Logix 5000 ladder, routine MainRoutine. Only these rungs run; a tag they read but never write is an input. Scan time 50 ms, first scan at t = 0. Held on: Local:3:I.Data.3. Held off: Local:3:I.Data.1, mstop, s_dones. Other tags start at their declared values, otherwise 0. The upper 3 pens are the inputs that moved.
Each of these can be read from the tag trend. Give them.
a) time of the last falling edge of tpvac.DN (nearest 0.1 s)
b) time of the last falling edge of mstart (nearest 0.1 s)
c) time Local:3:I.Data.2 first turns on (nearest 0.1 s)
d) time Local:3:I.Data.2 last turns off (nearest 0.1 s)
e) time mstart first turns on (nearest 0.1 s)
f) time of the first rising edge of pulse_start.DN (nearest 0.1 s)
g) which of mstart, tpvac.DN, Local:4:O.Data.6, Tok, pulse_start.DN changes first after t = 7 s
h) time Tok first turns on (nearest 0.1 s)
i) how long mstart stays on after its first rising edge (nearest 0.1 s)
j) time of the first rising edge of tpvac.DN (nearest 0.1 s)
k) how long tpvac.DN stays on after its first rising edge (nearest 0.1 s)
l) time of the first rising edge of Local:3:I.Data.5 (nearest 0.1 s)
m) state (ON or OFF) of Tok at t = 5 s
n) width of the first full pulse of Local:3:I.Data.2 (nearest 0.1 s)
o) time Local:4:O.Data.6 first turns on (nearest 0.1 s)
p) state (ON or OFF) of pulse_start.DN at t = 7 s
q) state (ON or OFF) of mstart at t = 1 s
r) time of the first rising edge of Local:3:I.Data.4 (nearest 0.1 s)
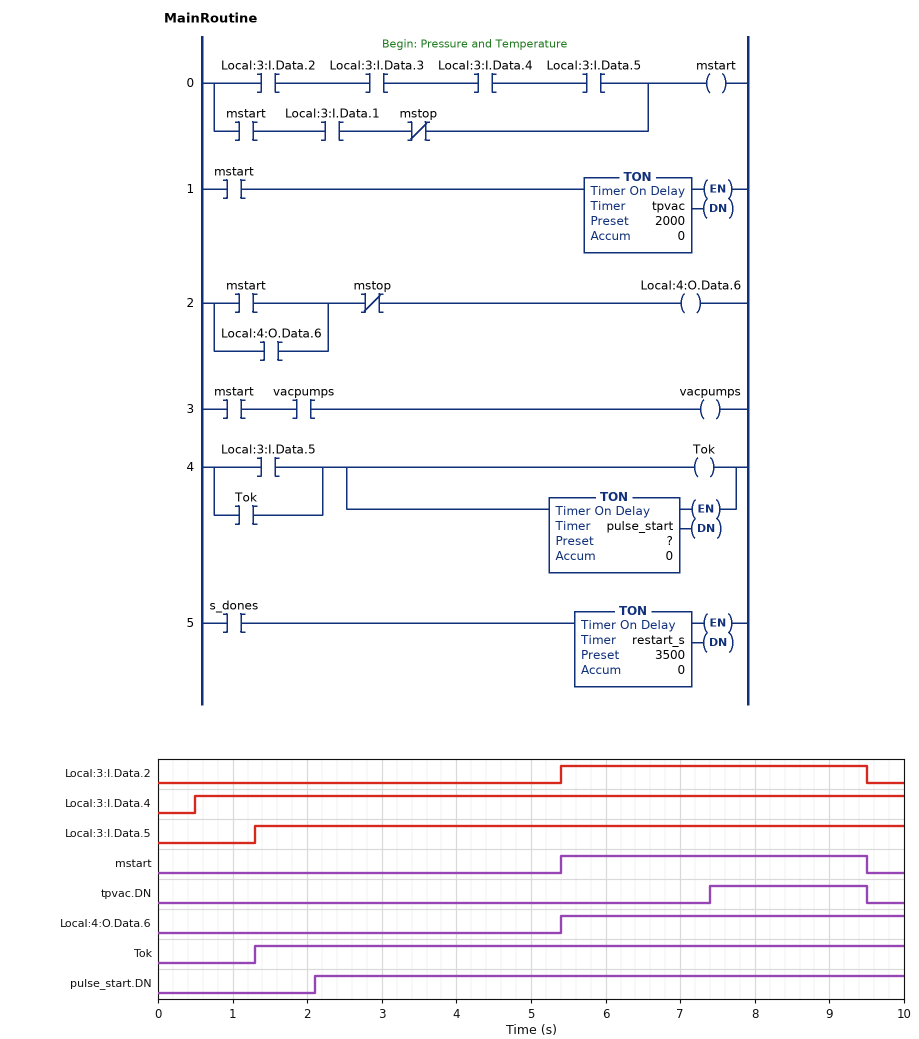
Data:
9.5 s
9.5 s
5.4 s
9.5 s
5.4 s
2.1 s
tpvac.DN
1.3 s
4.1 s
7.4 s
2.1 s
1.3 s
ON
4.1 s
5.4 s
ON
OFF
0.5 s
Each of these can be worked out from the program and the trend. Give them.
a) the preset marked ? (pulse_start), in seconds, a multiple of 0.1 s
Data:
0.8 s
